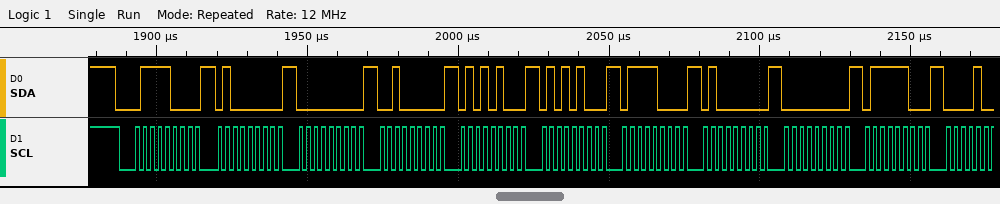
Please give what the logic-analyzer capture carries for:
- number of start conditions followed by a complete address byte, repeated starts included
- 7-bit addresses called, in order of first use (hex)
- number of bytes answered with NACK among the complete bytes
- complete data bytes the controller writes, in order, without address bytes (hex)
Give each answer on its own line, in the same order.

1
0x3C
0
40 00 20 54 54 78 40 00 7C
